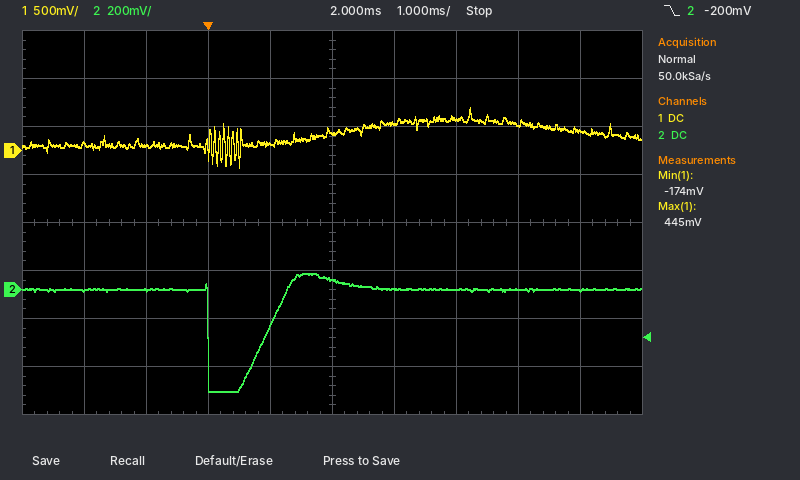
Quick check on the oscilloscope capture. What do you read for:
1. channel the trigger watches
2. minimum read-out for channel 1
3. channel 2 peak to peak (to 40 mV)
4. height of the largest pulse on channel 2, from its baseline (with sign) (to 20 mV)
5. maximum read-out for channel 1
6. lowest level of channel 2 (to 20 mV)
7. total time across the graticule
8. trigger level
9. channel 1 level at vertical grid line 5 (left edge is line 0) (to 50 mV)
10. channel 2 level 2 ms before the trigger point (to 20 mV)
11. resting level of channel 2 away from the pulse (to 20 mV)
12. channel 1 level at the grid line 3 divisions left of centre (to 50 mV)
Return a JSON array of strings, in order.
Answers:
["channel 2", "-174 mV", "480 mV", "-420 mV", "445 mV", "-420 mV", "10 ms", "-200 mV", "200 mV", "0 mV", "0 mV", "50 mV"]
